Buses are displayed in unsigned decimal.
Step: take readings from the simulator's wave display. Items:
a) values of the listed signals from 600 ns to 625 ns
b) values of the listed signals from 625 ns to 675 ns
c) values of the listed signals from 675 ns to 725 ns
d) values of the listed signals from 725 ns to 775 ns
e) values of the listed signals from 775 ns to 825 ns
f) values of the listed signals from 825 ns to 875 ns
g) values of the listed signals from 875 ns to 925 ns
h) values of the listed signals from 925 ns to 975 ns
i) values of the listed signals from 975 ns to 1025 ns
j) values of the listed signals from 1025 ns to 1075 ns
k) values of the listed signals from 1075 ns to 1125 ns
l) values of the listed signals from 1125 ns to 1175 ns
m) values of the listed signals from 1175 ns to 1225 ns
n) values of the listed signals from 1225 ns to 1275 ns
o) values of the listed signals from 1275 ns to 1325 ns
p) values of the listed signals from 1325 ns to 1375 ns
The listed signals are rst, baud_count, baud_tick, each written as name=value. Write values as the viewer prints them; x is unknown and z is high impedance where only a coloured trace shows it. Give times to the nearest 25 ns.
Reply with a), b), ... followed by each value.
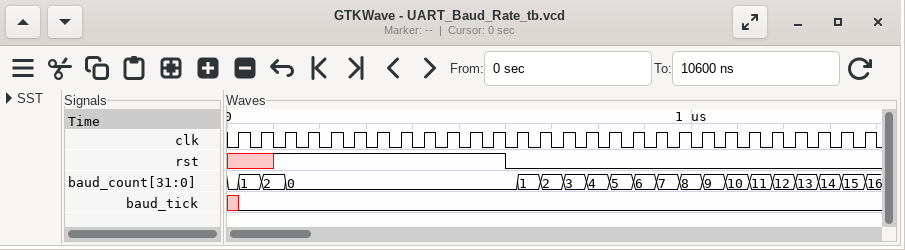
a) rst=0, baud_count=0, baud_tick=0
b) rst=0, baud_count=1, baud_tick=0
c) rst=0, baud_count=2, baud_tick=0
d) rst=0, baud_count=3, baud_tick=0
e) rst=0, baud_count=4, baud_tick=0
f) rst=0, baud_count=5, baud_tick=0
g) rst=0, baud_count=6, baud_tick=0
h) rst=0, baud_count=7, baud_tick=0
i) rst=0, baud_count=8, baud_tick=0
j) rst=0, baud_count=9, baud_tick=0
k) rst=0, baud_count=10, baud_tick=0
l) rst=0, baud_count=11, baud_tick=0
m) rst=0, baud_count=12, baud_tick=0
n) rst=0, baud_count=13, baud_tick=0
o) rst=0, baud_count=14, baud_tick=0
p) rst=0, baud_count=15, baud_tick=0
